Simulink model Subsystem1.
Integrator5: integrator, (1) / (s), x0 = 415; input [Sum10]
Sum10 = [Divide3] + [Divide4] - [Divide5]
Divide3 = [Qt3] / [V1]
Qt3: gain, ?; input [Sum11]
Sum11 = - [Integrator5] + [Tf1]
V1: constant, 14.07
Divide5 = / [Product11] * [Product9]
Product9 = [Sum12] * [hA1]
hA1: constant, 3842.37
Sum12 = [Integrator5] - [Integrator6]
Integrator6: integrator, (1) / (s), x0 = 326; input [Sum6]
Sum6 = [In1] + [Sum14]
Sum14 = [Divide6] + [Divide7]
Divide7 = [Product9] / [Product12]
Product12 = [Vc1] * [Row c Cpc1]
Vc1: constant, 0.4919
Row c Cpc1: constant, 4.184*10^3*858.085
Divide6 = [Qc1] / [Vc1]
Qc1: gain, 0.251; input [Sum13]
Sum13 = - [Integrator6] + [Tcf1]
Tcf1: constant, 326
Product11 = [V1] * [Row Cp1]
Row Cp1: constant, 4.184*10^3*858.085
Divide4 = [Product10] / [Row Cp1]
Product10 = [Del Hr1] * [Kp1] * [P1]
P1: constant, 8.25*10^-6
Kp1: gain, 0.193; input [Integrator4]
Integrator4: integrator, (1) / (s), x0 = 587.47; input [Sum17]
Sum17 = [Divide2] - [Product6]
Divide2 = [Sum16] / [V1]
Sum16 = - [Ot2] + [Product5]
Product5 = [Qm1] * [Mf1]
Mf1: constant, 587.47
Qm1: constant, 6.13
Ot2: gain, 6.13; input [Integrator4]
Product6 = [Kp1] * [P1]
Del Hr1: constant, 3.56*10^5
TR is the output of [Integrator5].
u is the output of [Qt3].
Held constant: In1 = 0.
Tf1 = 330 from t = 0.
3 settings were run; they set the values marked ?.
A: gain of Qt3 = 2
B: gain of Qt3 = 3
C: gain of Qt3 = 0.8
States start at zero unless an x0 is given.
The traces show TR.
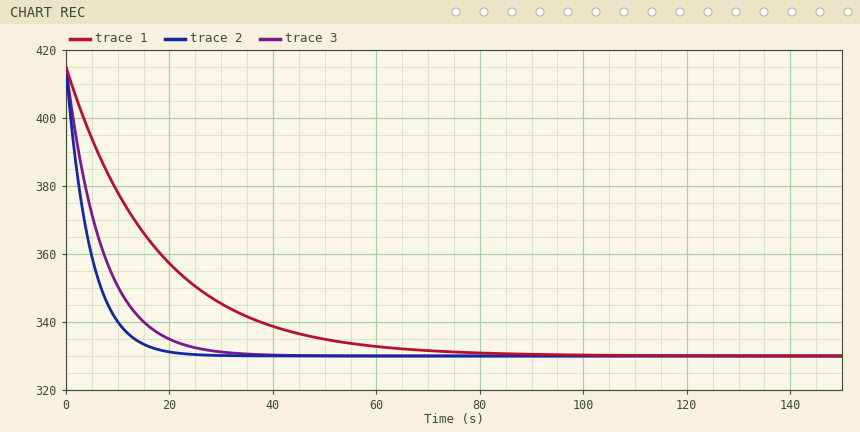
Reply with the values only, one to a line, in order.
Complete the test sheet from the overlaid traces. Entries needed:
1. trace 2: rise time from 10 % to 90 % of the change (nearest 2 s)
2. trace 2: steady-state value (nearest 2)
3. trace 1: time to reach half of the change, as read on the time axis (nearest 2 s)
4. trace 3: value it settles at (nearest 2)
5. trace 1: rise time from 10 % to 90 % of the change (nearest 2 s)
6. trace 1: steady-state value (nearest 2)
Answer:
10 s
330
12 s
330
38 s
330
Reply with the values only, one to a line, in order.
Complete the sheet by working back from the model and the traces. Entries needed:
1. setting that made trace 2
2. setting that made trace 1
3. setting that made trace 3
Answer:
B
C
A
